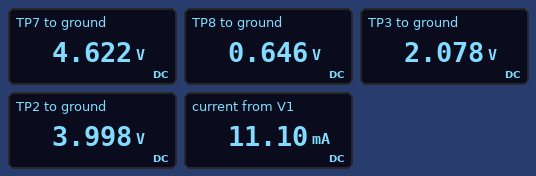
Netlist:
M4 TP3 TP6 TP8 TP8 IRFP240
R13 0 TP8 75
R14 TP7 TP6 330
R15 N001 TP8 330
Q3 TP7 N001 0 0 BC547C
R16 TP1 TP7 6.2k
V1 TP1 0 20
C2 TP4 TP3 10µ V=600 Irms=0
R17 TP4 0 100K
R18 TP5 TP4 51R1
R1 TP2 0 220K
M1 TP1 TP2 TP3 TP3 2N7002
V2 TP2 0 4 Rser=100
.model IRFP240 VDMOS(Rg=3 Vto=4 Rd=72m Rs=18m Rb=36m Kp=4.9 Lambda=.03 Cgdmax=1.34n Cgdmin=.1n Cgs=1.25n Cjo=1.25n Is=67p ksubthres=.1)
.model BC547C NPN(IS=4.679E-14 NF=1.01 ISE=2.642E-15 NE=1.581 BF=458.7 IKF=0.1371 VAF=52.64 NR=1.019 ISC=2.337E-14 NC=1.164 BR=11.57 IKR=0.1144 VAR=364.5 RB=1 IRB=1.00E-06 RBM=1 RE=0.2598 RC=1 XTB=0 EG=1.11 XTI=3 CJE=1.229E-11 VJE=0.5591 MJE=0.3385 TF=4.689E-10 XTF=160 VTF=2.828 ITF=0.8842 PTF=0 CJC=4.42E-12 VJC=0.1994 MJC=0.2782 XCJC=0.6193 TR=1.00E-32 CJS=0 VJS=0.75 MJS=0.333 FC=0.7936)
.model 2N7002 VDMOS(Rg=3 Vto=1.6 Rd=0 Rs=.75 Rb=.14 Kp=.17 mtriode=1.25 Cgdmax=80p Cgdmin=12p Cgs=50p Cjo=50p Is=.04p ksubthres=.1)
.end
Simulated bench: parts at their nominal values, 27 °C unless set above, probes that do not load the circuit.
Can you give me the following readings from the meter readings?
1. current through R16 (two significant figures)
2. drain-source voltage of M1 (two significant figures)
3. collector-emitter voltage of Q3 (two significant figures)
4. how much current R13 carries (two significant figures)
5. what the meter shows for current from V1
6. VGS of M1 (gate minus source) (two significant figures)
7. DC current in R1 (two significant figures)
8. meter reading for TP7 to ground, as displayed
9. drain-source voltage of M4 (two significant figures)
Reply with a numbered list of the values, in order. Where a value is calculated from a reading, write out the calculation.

1. (20 V - 4.622 V) / 6.2 kΩ = 2.5 mA
2. 20 V - 2.078 V = 18 V
3. 4.622 V = 4.6 V
4. (646 mV) / 75 Ω = 8.6 mA
5. 11.10 mA
6. 3.998 V - 2.078 V = 1.9 V
7. (3.998 V) / 220 kΩ = 18 µA
8. 4.622 V
9. 2.078 V - 646 mV = 1.4 V
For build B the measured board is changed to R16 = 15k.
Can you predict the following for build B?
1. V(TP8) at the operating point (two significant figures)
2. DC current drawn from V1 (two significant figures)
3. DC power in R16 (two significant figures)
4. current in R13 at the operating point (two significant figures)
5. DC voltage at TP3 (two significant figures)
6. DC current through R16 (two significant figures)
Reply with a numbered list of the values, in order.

1. 620 mV
2. 9.3 mA
3. 16 mW
4. 8.3 mA
5. 2.1 V
6. 1.0 mA
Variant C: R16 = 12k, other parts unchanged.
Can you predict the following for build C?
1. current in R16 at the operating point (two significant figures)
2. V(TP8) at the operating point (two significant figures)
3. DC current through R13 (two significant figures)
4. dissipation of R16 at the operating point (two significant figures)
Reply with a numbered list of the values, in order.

1. 1.3 mA
2. 630 mV
3. 8.4 mA
4. 20 mW
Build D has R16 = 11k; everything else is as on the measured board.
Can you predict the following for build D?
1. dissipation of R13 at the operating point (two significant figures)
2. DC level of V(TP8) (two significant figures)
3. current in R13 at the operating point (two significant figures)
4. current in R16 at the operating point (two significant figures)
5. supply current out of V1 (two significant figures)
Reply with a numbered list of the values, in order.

1. 5.3 mW
2. 630 mV
3. 8.4 mA
4. 1.4 mA
5. 9.8 mA
